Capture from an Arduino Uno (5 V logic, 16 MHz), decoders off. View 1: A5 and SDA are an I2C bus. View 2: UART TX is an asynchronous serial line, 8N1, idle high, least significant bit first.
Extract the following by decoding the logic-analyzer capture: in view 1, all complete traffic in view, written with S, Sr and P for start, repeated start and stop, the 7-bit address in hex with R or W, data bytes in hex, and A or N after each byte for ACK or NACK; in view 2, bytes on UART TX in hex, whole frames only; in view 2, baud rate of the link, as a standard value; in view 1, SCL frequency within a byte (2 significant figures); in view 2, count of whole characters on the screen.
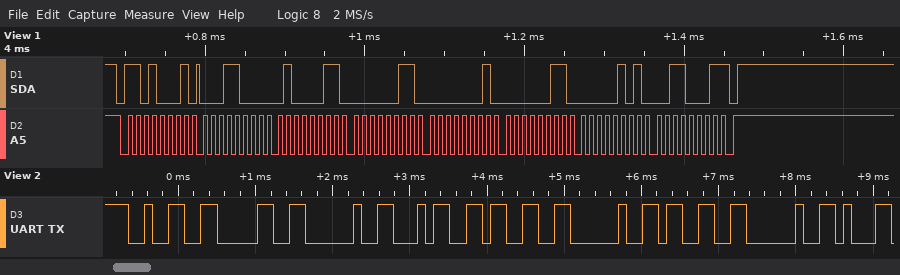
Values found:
S 68R A 18 A 43 A 03 A 01 A 03 A 05 A 31 N P
32 30 20 34 33 20 33 20
9600 baud
100 kHz
8
